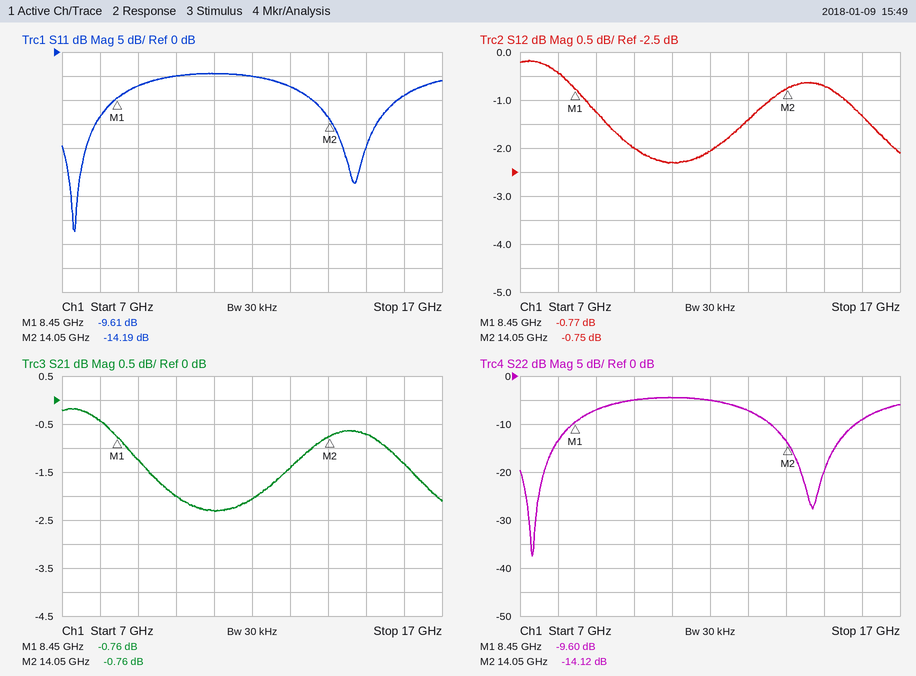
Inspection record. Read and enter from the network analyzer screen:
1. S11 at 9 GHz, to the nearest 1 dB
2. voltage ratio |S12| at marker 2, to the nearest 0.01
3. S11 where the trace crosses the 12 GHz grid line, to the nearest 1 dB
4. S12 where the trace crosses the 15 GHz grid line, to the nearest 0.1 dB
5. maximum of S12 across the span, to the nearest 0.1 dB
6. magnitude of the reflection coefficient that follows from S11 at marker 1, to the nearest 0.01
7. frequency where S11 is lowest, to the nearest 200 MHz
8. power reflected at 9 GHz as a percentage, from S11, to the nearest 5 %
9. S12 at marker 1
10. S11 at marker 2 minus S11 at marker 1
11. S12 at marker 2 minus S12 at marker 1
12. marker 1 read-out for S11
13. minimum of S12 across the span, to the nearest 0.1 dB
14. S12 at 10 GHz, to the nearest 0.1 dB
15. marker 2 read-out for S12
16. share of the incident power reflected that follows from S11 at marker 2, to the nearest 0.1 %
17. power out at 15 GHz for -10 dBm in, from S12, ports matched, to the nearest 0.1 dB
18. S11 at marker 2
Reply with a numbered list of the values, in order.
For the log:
1. -7 dB
2. 0.92
3. -5 dB
4. -0.7 dB
5. -0.2 dB
6. 0.33
7. 7.4 GHz
8. 20 %
9. -0.77 dB
10. -4.58 dB
11. 0.02 dB
12. -9.61 dB
13. -2.3 dB
14. -2.0 dB
15. -0.75 dB
16. 3.8 %
17. -10.7 dBm
18. -14.19 dB
